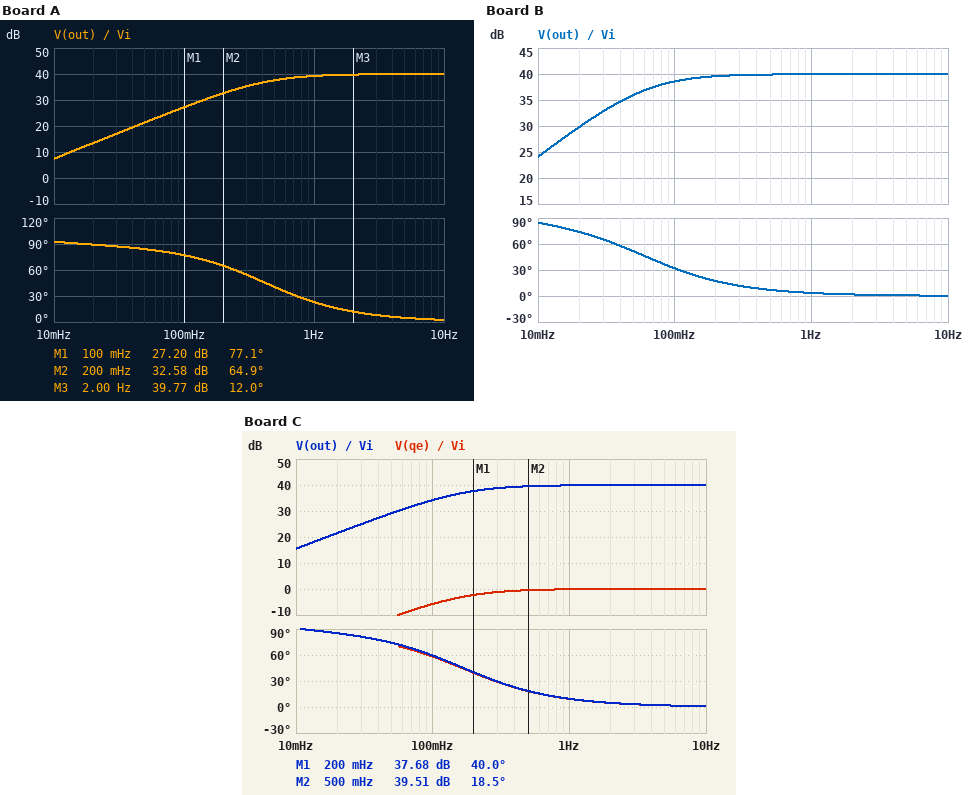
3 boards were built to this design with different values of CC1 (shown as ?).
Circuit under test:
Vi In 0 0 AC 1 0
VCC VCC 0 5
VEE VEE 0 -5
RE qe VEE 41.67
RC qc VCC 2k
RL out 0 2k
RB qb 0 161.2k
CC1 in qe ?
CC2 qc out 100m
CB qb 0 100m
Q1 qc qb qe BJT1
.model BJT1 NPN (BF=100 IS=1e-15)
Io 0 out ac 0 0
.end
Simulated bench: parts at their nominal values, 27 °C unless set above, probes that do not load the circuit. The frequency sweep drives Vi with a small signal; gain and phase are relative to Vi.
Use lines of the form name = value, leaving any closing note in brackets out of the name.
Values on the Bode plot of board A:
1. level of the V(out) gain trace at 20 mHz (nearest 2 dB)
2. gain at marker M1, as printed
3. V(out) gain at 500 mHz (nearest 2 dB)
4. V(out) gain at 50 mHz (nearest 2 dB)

level of the V(out) gain trace at 20 mHz = 14 dB
gain at marker M1, as printed = 27.20 dB
V(out) gain at 500 mHz = 38 dB
V(out) gain at 50 mHz = 22 dB
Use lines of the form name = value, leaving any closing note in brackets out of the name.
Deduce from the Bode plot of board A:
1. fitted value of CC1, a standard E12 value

fitted value of CC1, a standard E12 value = 47 mF
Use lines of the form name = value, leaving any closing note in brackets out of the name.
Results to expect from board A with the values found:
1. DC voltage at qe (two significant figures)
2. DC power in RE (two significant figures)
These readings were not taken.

DC voltage at qe = -4.9 V
DC power in RE = 280 µW
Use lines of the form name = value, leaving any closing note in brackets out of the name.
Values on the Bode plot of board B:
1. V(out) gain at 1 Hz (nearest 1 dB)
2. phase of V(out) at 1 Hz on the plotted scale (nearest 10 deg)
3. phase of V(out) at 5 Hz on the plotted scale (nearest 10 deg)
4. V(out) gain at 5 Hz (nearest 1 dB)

V(out) gain at 1 Hz = 40 dB
phase of V(out) at 1 Hz on the plotted scale = 0 deg
phase of V(out) at 5 Hz on the plotted scale = 0 deg
V(out) gain at 5 Hz = 40 dB
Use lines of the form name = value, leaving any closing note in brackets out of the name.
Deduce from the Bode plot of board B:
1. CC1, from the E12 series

CC1, from the E12 series = 330 mF
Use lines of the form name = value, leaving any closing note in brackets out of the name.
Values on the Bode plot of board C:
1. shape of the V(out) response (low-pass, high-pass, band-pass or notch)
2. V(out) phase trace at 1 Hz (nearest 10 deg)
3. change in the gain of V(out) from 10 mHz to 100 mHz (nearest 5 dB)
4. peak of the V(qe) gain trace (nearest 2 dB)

shape of the V(out) response = high-pass
V(out) phase trace at 1 Hz = 10 deg
change in the gain of V(out) from 10 mHz to 100 mHz = 20 dB
peak of the V(qe) gain trace = 0 dB
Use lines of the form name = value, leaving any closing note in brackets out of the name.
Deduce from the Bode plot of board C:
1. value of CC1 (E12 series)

value of CC1 = 120 mF
